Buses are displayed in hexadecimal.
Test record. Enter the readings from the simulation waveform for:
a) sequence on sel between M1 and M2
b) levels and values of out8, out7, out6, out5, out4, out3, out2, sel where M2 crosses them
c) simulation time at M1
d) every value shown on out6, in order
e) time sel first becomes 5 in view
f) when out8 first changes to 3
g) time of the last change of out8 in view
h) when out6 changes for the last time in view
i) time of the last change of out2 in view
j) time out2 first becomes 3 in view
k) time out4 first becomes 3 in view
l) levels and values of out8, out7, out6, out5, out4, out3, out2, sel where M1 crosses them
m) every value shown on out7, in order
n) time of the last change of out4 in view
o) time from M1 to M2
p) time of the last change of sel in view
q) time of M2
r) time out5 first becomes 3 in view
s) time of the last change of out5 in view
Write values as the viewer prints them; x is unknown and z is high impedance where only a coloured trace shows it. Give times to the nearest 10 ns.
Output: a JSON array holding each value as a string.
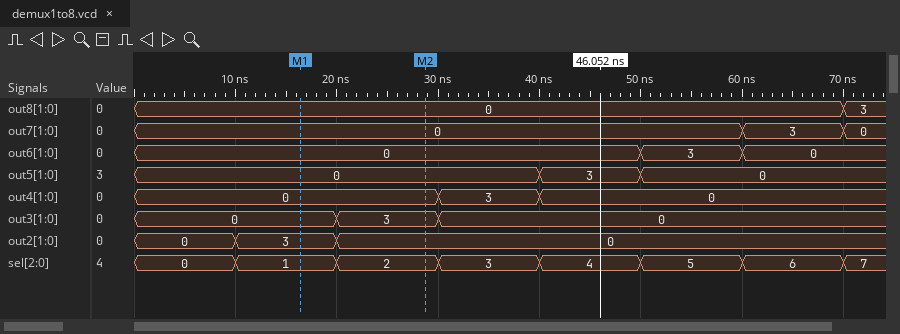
["1, 2", "out8=0, out7=0, out6=0, out5=0, out4=0, out3=3, out2=0, sel=2", "20 ns", "0, 3, 0", "50 ns", "70 ns", "70 ns", "60 ns", "20 ns", "10 ns", "30 ns", "out8=0, out7=0, out6=0, out5=0, out4=0, out3=0, out2=3, sel=1", "0, 3, 0", "40 ns", "10 ns", "70 ns", "30 ns", "40 ns", "50 ns"]
